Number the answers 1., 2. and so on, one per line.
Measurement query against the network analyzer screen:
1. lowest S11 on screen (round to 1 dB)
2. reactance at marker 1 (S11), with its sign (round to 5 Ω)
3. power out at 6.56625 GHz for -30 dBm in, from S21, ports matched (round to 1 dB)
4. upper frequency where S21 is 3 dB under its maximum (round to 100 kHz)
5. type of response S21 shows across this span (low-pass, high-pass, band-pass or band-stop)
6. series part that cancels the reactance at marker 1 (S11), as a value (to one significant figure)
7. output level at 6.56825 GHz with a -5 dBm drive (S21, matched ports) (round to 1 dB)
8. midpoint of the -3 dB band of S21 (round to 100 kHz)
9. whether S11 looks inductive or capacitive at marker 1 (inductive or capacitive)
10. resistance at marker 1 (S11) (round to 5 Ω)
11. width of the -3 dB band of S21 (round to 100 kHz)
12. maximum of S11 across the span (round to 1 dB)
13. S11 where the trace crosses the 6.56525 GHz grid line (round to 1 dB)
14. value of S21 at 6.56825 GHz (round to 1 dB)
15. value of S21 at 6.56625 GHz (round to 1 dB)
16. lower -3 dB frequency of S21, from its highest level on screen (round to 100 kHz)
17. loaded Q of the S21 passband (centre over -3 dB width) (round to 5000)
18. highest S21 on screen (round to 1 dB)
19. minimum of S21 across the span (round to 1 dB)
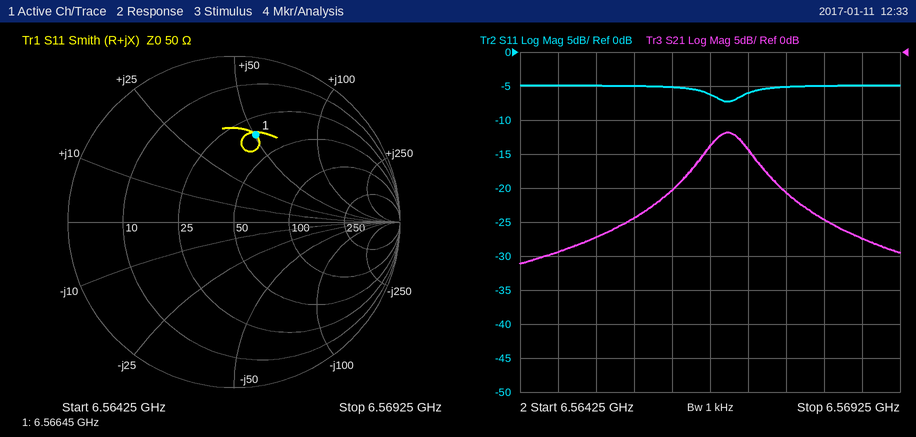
1. -7 dB
2. +50 Ω
3. -50 dBm
4. 6.5673 GHz
5. band-pass
6. 500 fF
7. -30 dBm
8. 6.5670 GHz
9. inductive
10. 35 Ω
11. 600 kHz
12. -5 dB
13. -5 dB
14. -25 dB
15. -20 dB
16. 6.5667 GHz
17. 10000
18. -12 dB
19. -31 dB
